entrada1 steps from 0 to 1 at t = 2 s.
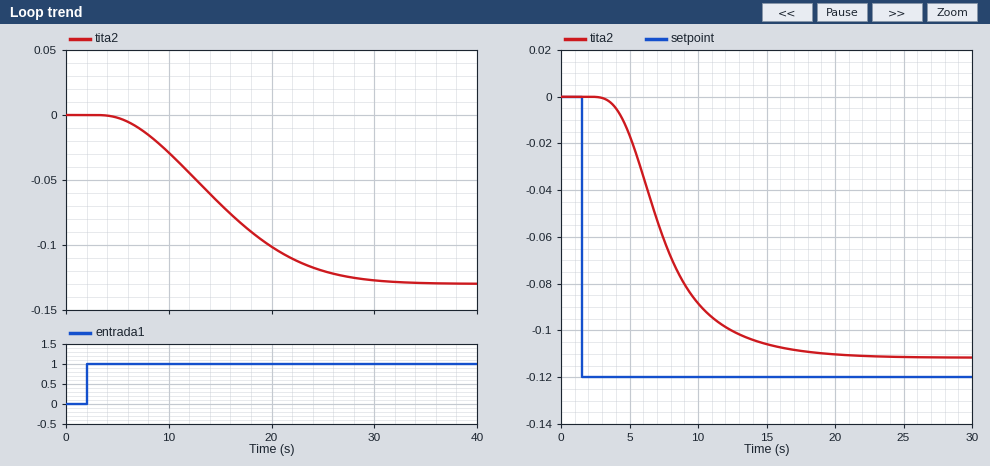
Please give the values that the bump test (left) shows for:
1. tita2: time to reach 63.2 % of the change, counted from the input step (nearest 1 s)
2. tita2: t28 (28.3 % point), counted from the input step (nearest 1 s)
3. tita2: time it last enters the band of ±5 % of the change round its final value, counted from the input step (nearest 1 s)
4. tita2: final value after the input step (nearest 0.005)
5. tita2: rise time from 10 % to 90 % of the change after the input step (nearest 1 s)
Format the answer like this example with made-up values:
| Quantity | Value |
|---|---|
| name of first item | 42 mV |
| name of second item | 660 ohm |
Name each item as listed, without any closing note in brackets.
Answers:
| Quantity | Value |
|---|---|
| tita2: time to reach 63.2 % of the change, counted from the input step | 15 s |
| tita2: t28 (28.3 % point), counted from the input step | 9 s |
| tita2: time it last enters the band of ±5 % of the change round its final value, counted from the input step | 25 s |
| tita2: final value after the input step | -0.130 |
| tita2: rise time from 10 % to 90 % of the change after the input step | 16 s |
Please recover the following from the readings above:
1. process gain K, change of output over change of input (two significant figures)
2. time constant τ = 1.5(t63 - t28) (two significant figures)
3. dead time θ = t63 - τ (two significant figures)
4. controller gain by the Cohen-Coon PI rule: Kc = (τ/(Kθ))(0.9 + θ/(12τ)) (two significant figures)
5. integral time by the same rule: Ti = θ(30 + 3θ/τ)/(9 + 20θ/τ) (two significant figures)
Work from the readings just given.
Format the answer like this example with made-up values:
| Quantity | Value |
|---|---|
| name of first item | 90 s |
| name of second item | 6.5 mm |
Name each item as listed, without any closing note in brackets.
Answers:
| Quantity | Value |
|---|---|
| process gain K, change of output over change of input | -0.13 |
| time constant τ = 1.5(t63 - t28) | 9.0 s |
| dead time θ = t63 - τ | 6.0 s |
| controller gain by the Cohen-Coon PI rule: Kc = (τ/(Kθ))(0.9 + θ/(12τ)) | -11 |
| integral time by the same rule: Ti = θ(30 + 3θ/τ)/(9 + 20θ/τ) | 8.6 s |
